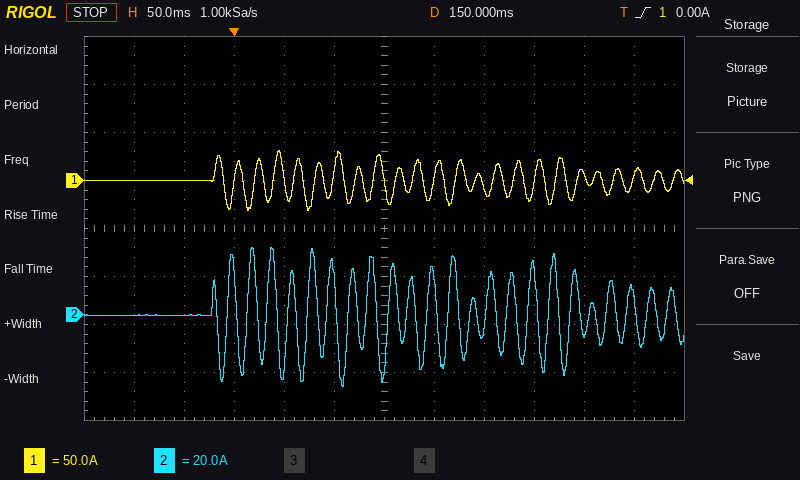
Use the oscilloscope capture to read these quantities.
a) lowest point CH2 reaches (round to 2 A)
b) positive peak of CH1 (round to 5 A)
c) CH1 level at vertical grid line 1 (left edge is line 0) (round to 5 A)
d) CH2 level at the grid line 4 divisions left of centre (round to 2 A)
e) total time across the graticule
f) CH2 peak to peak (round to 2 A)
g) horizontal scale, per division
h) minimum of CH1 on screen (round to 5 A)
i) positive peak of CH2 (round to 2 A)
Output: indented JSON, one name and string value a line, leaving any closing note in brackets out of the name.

{
  "lowest point CH2 reaches": "-30 A",
  "positive peak of CH1": "30 A",
  "CH1 level at vertical grid line 1 (left edge is line 0)": "0 A",
  "CH2 level at the grid line 4 divisions left of centre": "0 A",
  "total time across the graticule": "600 ms",
  "CH2 peak to peak": "58 A",
  "horizontal scale, per division": "50 ms",
  "minimum of CH1 on screen": "-30 A",
  "positive peak of CH2": "28 A"
}
